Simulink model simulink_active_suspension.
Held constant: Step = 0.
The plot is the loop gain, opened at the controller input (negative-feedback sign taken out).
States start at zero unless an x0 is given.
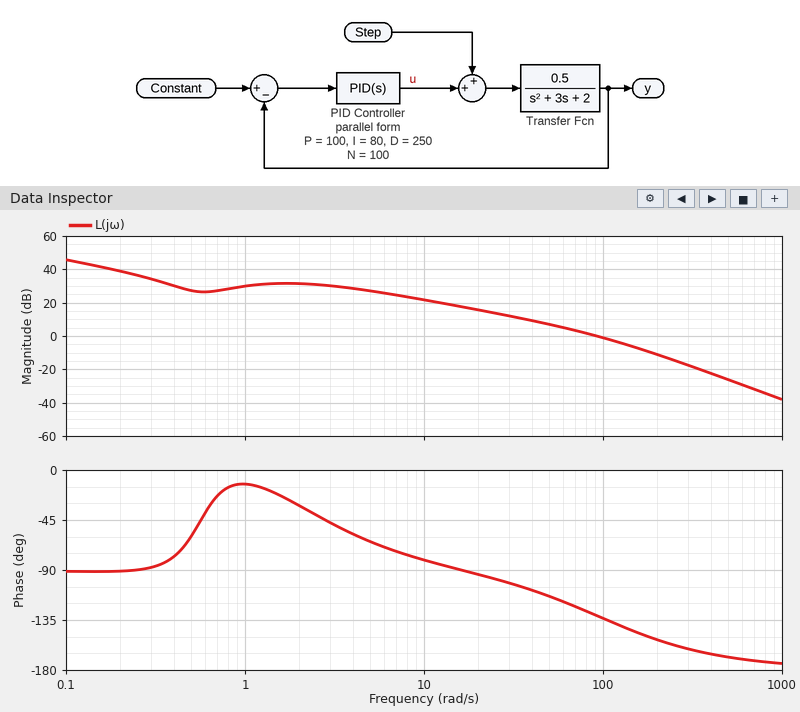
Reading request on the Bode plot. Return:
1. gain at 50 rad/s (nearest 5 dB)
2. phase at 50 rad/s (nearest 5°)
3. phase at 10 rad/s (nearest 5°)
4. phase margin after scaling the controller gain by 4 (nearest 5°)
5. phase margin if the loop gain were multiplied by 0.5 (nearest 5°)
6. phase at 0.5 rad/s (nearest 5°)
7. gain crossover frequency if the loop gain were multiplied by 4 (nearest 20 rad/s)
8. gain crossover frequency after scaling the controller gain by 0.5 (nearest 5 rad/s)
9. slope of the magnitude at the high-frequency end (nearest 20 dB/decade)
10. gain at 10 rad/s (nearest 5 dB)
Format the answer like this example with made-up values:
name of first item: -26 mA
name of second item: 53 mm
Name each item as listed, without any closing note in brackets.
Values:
gain at 50 rad/s: 5 dB
phase at 50 rad/s: -115°
phase at 10 rad/s: -80°
phase margin after scaling the controller gain by 4: 25°
phase margin if the loop gain were multiplied by 0.5: 65°
phase at 0.5 rad/s: -60°
gain crossover frequency if the loop gain were multiplied by 4: 220 rad/s
gain crossover frequency after scaling the controller gain by 0.5: 55 rad/s
slope of the magnitude at the high-frequency end: -40 dB/decade
gain at 10 rad/s: 20 dB
